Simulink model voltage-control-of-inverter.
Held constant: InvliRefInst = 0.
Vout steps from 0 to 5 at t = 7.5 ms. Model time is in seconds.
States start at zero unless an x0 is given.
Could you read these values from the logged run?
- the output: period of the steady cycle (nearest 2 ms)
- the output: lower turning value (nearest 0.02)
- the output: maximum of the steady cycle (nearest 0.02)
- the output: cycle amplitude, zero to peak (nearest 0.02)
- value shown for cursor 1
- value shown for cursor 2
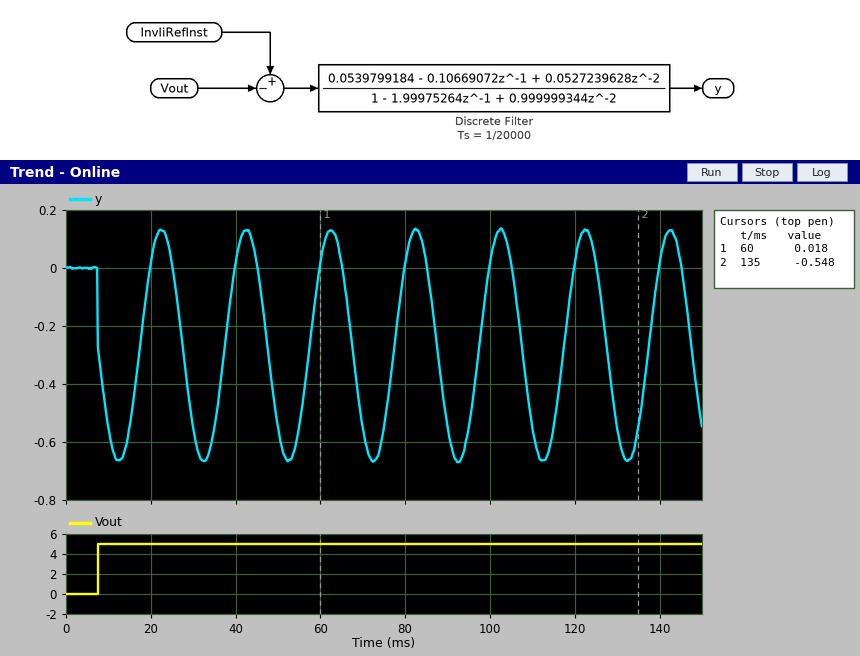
20 ms
-0.66
0.14
0.40
0.018
-0.548
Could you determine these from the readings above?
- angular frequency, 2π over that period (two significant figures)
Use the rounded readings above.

0.31 rad/ms
